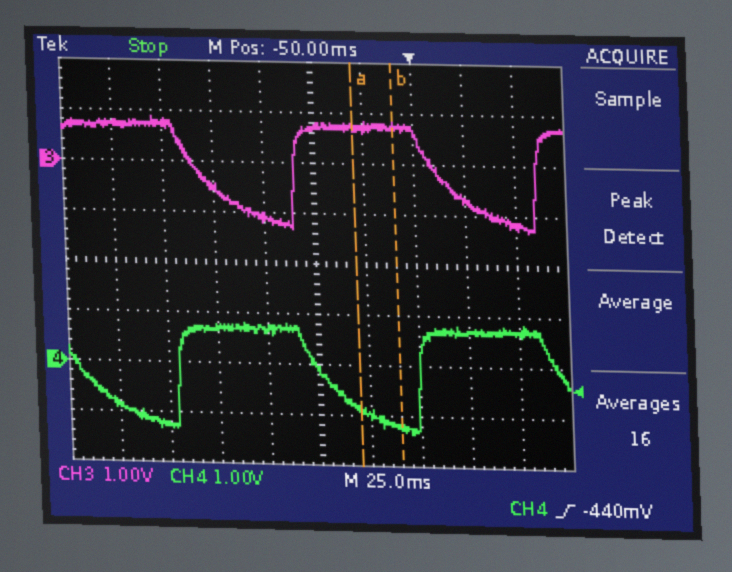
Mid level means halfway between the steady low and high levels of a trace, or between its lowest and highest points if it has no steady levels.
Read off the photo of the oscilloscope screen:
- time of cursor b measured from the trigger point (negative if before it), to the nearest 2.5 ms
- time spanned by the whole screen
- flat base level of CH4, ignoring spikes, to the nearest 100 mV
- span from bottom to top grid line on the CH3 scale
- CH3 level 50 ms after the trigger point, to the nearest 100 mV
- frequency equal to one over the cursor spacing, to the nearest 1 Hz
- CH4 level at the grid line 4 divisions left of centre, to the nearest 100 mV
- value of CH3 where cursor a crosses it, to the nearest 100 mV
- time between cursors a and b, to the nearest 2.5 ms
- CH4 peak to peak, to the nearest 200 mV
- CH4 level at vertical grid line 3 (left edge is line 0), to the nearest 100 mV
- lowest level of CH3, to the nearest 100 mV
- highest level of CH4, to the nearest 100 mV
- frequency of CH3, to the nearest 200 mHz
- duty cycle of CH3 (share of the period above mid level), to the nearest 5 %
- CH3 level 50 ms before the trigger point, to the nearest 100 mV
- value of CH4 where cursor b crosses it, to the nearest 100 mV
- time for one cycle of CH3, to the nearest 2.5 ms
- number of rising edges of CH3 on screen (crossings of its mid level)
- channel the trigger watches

-10.0 ms
250 ms
-1.2 V
8 V
-1.2 V
50 Hz
-800 mV
700 mV
20.0 ms
2.2 V
700 mV
-1.3 V
800 mV
8.4 Hz
60 %
700 mV
-1.2 V
120.0 ms
2
CH4
